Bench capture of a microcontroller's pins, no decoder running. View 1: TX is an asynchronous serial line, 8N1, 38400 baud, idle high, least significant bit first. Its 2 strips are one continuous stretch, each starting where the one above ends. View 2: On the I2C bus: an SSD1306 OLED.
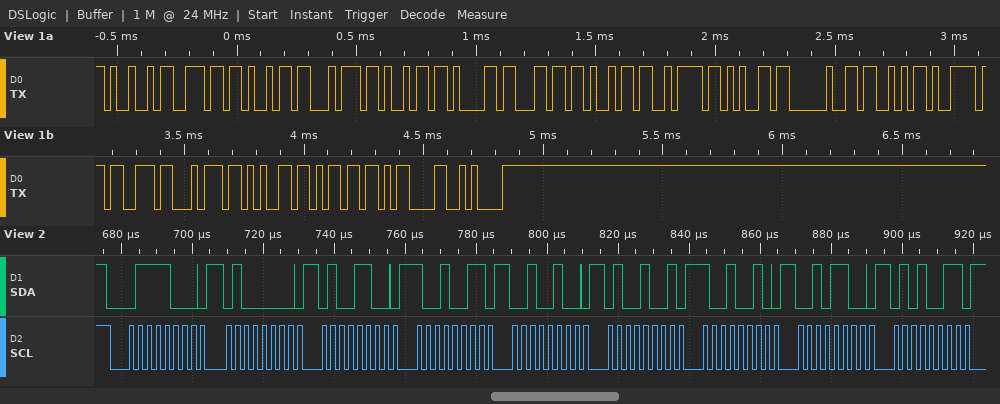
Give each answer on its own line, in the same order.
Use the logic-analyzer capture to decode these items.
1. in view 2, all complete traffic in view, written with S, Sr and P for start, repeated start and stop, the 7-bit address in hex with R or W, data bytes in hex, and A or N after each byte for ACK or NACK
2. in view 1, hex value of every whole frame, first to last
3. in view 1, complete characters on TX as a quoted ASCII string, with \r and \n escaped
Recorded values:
S 3CW A 40 A 4C A 93 A 24 A 49 A 92 A 2C A 53 A
49 6E 69 74 69 61 6C 69 7A 65 20 53 79 73 74 65 6D 0D 0A
"Initialize System\r\n"
